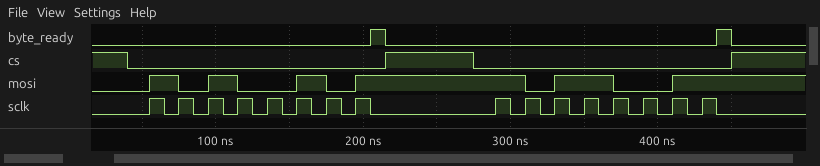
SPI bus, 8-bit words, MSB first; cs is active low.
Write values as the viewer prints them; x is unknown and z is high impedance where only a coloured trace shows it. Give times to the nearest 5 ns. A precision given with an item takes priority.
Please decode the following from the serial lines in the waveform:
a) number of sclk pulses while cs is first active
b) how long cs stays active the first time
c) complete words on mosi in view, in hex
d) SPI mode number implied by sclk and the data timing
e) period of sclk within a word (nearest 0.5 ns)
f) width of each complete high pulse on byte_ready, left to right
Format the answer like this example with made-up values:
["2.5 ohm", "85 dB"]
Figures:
["8", "175 ns", "A5, B3", "1", "20 ns", "10 ns, 10 ns"]
